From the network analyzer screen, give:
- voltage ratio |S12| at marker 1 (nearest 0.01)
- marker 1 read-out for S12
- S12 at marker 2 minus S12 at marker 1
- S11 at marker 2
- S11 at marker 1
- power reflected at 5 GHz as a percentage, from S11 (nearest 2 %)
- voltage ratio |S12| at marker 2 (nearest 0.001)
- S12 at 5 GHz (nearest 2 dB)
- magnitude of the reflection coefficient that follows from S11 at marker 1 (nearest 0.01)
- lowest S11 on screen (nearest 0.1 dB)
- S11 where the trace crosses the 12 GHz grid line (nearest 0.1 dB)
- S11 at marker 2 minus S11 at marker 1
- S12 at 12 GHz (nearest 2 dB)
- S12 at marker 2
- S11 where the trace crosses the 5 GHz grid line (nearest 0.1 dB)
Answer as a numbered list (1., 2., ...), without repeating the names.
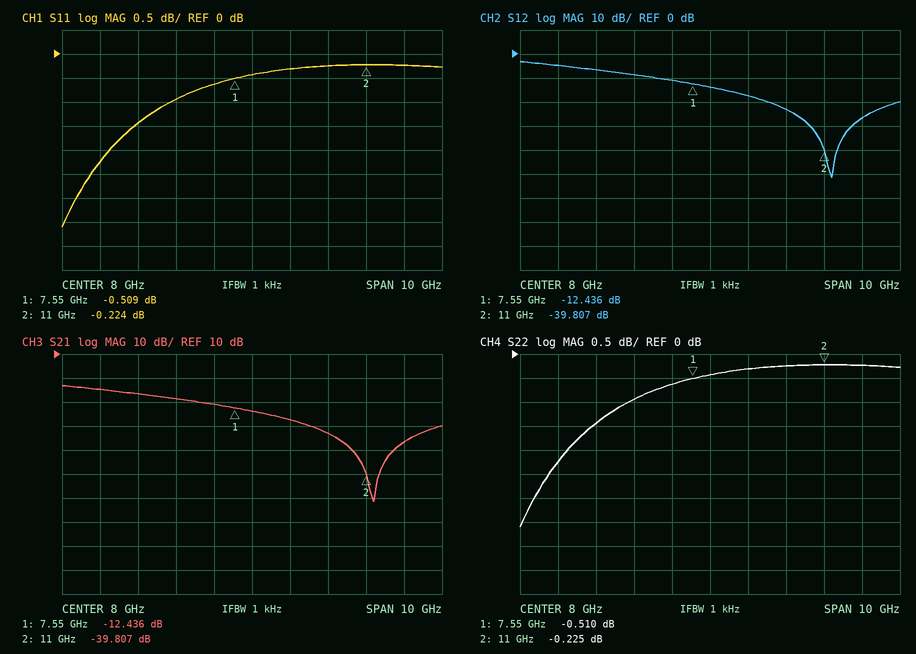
1. 0.24
2. -12.436 dB
3. -27.371 dB
4. -0.224 dB
5. -0.509 dB
6. 72 %
7. 0.010
8. -6 dB
9. 0.94
10. -3.6 dB
11. -0.2 dB
12. 0.285 dB
13. -26 dB
14. -39.807 dB
15. -1.4 dB
